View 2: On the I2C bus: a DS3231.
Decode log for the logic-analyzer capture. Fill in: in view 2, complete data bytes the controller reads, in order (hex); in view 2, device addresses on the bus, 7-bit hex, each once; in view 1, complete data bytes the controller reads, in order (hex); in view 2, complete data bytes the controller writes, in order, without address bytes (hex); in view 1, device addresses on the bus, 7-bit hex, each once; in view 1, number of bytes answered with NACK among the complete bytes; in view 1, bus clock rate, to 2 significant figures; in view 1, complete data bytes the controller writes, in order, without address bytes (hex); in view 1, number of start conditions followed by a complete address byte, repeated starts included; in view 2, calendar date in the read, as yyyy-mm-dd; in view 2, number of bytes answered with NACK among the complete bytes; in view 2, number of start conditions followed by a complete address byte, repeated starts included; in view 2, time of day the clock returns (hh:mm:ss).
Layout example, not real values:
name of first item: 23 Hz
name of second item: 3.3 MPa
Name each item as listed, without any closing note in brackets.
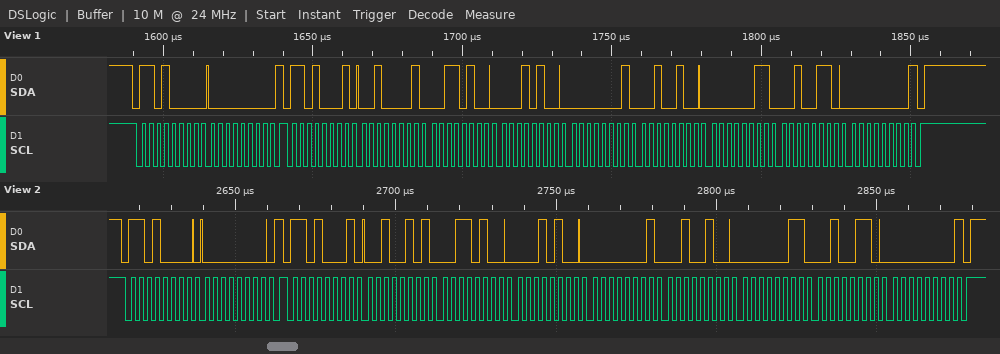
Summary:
in view 2, complete data bytes the controller reads, in order: 25 34 14 01 24 03 26 00
in view 2, device addresses on the bus, 7-bit hex, each once: 0x68
in view 1, complete data bytes the controller reads, in order: 21 34 14 01 24 03 26 00
in view 2, complete data bytes the controller writes, in order, without address bytes: 00
in view 1, device addresses on the bus, 7-bit hex, each once: 0x68
in view 1, number of bytes answered with NACK among the complete bytes: 1
in view 1, bus clock rate, to 2 significant figures: 400 kHz
in view 1, complete data bytes the controller writes, in order, without address bytes: 00
in view 1, number of start conditions followed by a complete address byte, repeated starts included: 2
in view 2, calendar date in the read, as yyyy-mm-dd: 2026-03-24
in view 2, number of bytes answered with NACK among the complete bytes: 1
in view 2, number of start conditions followed by a complete address byte, repeated starts included: 2
in view 2, time of day the clock returns: 14:34:25
